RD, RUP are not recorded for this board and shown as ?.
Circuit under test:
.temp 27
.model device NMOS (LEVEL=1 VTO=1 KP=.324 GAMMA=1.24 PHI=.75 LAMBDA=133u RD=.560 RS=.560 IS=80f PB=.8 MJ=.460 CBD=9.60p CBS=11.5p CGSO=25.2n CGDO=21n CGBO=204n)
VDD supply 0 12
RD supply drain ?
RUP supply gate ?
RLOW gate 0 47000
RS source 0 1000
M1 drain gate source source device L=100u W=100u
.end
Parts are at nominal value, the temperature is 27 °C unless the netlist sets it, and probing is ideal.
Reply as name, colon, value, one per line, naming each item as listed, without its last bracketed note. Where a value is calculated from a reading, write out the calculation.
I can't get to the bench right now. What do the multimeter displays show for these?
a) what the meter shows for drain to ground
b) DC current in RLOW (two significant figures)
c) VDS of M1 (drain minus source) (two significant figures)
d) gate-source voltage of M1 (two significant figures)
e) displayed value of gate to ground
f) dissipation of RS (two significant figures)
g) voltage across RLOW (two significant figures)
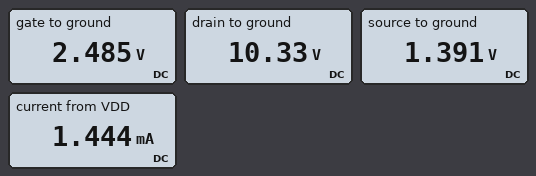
what the meter shows for drain to ground: 10.33 V
DC current in RLOW: (2.485 V) / 47 kΩ = 53 µA
VDS of M1 (drain minus source): 10.33 V - 1.391 V = 8.9 V
gate-source voltage of M1: 2.485 V - 1.391 V = 1.1 V
displayed value of gate to ground: 2.485 V
dissipation of RS: (1.391 V)^2 / 1 kΩ = 1.9 mW
voltage across RLOW: 2.485 V = 2.5 V
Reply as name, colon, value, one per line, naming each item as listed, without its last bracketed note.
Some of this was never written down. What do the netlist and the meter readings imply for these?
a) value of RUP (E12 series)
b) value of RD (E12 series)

value of RUP: 180 kΩ
value of RD: 1.2 kΩ
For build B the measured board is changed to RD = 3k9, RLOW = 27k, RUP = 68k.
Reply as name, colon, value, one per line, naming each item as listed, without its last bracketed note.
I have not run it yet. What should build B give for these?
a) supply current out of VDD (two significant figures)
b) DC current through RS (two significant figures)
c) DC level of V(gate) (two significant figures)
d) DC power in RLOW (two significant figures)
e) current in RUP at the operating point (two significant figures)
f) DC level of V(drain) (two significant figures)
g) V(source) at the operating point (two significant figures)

supply current out of VDD: 2.4 mA
DC current through RS: 2.3 mA
DC level of V(gate): 3.4 V
DC power in RLOW: 430 µW
current in RUP at the operating point: 130 µA
DC level of V(drain): 3.1 V
V(source) at the operating point: 2.3 V
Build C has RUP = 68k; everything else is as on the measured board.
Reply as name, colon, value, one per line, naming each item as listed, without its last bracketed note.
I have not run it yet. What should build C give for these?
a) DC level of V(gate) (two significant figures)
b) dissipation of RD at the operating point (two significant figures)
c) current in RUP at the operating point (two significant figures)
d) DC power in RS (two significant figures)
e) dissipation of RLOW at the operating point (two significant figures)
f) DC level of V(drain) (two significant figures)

DC level of V(gate): 4.9 V
dissipation of RD at the operating point: 17 mW
current in RUP at the operating point: 100 µA
DC power in RS: 14 mW
dissipation of RLOW at the operating point: 510 µW
DC level of V(drain): 7.5 V
